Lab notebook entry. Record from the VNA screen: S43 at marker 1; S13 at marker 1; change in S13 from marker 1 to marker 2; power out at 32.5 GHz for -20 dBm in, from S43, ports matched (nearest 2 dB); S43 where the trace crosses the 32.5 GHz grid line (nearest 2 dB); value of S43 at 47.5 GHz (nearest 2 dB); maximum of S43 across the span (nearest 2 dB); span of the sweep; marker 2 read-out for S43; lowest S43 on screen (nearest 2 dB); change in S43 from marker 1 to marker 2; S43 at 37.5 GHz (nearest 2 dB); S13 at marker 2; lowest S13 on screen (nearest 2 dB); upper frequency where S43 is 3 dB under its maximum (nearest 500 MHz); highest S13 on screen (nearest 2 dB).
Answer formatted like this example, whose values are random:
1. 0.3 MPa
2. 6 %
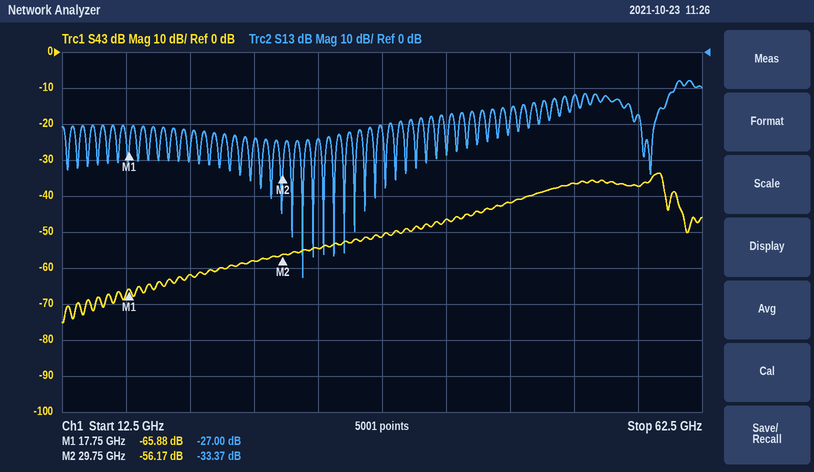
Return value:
1. -65.88 dB
2. -27.00 dB
3. -6.37 dB
4. -74 dBm
5. -54 dB
6. -42 dB
7. -34 dB
8. 50 GHz
9. -56.17 dB
10. -76 dB
11. 9.71 dB
12. -52 dB
13. -33.37 dB
14. -62 dB
15. 59.5 GHz
16. -8 dB
